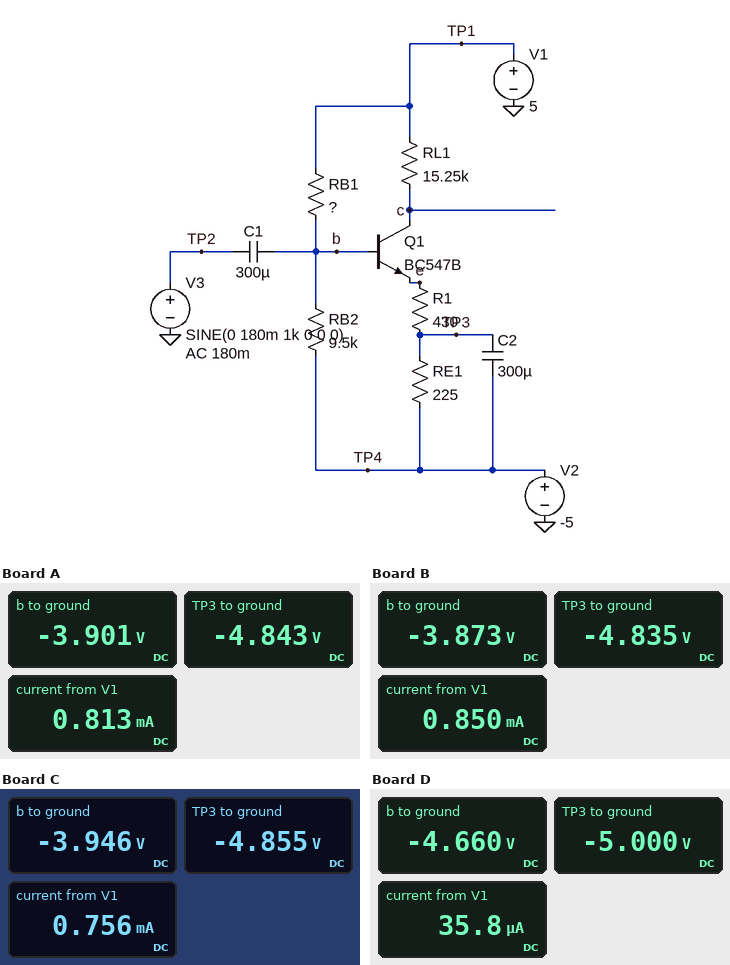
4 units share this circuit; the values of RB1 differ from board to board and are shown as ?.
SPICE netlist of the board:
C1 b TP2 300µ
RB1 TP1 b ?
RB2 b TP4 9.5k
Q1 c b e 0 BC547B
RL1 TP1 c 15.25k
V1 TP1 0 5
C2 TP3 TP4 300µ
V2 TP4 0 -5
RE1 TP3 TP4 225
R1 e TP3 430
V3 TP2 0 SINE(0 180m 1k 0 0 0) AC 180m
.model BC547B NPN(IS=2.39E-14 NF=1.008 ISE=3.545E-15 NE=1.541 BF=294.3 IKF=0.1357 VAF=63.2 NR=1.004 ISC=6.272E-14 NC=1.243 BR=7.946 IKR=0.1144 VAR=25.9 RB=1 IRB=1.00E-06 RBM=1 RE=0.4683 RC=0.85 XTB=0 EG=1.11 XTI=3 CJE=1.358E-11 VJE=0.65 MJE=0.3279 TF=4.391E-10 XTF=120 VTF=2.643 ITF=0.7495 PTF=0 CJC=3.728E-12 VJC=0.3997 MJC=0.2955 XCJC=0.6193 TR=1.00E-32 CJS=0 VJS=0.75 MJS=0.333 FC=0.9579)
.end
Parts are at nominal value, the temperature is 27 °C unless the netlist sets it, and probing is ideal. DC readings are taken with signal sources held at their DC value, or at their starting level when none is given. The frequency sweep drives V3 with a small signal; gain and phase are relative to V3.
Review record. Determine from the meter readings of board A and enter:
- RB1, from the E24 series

47 kΩ
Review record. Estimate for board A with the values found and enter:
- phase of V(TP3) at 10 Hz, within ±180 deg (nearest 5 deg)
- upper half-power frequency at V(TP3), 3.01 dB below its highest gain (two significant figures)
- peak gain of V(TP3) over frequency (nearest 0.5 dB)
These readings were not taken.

-65 deg
4.7 Hz
-13.5 dB
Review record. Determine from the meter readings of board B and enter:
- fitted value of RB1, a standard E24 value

39 kΩ
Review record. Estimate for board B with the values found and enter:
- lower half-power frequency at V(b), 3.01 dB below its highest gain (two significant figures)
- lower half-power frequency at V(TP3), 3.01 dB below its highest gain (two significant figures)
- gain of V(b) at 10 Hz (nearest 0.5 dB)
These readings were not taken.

840 mHz
520 mHz
0 dB
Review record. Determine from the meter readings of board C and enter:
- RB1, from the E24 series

68 kΩ
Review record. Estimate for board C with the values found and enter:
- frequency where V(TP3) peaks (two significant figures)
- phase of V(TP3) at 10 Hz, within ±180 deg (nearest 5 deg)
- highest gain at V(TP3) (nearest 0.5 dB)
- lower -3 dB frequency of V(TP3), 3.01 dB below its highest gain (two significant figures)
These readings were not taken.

1.4 Hz
-70 deg
-14.0 dB
450 mHz
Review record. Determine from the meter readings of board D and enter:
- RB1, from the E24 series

270 kΩ
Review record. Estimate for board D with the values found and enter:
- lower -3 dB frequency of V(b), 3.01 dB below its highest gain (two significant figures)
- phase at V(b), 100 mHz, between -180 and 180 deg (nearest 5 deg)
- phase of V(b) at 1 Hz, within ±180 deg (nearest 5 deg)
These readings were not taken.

58 mHz
30 deg
5 deg
